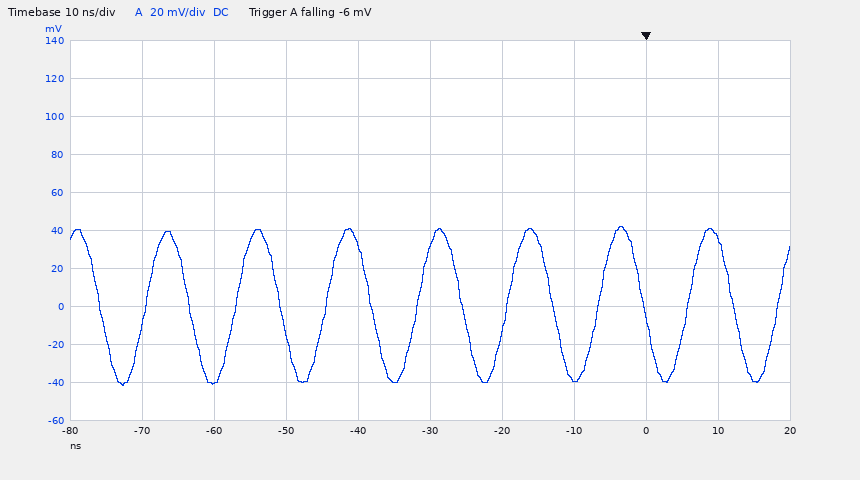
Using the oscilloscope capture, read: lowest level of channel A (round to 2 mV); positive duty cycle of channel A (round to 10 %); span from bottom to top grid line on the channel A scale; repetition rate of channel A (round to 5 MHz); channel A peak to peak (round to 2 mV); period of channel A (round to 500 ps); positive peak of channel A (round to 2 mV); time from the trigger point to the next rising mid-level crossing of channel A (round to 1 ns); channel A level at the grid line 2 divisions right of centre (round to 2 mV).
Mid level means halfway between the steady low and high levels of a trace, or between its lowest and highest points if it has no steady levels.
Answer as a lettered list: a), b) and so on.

a) -42 mV
b) 50 %
c) 200 mV
d) 80 MHz
e) 84 mV
f) 12.5 ns
g) 42 mV
h) 6 ns
i) -38 mV
